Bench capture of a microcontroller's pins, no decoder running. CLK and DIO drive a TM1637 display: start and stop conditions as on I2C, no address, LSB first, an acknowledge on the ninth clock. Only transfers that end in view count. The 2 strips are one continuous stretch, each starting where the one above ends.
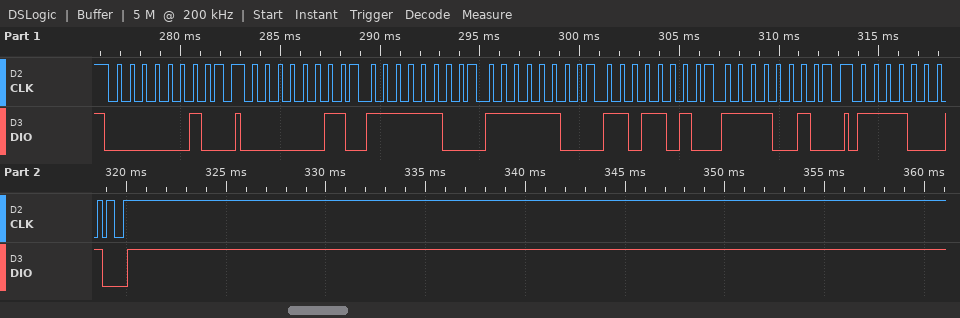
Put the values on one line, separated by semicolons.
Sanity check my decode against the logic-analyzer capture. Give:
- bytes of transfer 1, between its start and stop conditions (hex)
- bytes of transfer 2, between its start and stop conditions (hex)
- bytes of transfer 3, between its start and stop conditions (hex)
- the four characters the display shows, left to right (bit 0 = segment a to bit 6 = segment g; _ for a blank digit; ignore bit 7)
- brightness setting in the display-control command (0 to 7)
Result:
40; C0 3F 3F 5B 4F; 8F; 0023; 7
